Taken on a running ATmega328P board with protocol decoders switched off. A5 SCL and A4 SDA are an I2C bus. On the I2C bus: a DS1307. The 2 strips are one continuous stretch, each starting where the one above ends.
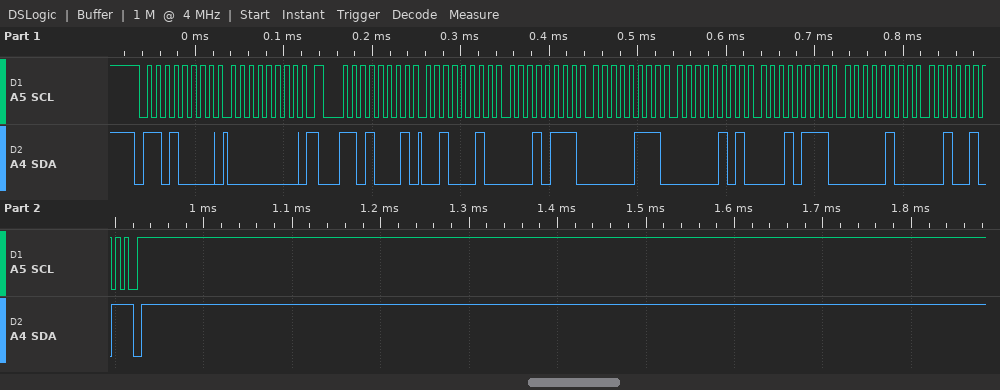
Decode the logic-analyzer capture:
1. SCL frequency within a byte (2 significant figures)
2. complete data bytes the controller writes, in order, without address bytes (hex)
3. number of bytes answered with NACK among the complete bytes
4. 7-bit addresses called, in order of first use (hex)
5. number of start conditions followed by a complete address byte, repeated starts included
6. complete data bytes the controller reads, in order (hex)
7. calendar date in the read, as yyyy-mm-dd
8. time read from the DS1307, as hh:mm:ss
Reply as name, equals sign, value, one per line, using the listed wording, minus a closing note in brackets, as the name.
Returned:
SCL frequency within a byte = 100 kHz
complete data bytes the controller writes, in order, without address bytes = 00
number of bytes answered with NACK among the complete bytes = 1
7-bit addresses called, in order of first use = 0x68
number of start conditions followed by a complete address byte, repeated starts included = 2
complete data bytes the controller reads, in order = 22 17 07 05 17 04 25
calendar date in the read, as yyyy-mm-dd = 2025-04-17
time read from the DS1307, as hh:mm:ss = 07:17:22
